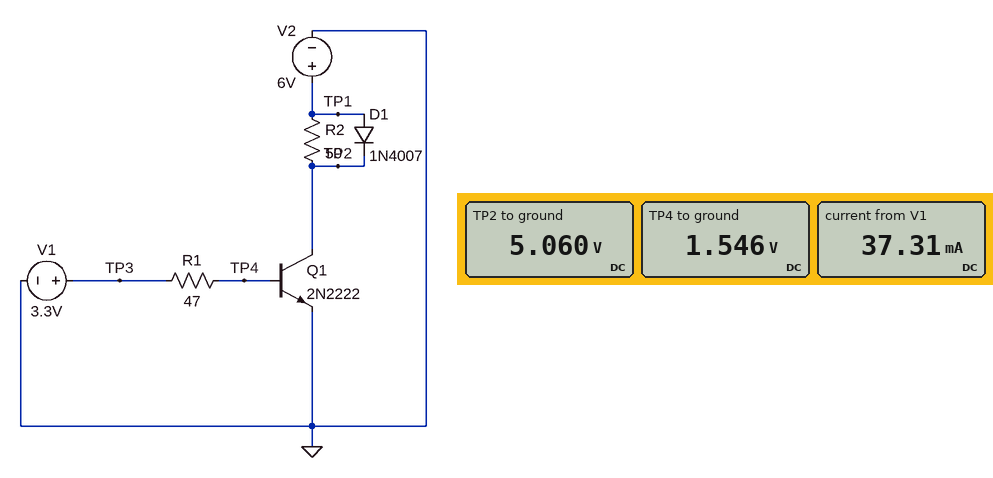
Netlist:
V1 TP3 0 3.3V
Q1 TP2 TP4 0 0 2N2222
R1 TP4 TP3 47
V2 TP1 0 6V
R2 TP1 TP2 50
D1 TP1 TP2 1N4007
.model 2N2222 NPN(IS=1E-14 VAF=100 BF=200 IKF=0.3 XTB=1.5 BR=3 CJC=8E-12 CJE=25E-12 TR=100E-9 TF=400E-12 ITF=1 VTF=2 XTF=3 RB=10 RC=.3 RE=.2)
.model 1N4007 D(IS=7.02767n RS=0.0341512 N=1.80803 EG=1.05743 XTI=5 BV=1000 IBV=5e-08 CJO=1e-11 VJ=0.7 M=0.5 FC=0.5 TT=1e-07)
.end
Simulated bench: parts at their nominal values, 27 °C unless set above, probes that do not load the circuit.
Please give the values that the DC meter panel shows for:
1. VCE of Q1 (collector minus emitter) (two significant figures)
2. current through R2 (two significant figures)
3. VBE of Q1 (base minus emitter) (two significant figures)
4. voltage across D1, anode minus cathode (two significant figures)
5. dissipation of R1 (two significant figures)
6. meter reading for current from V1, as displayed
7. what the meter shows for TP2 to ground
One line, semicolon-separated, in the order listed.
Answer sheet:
5.1 V; 19 mA; 1.5 V; 940 mV; 65 mW; 37.31 mA; 5.060 V
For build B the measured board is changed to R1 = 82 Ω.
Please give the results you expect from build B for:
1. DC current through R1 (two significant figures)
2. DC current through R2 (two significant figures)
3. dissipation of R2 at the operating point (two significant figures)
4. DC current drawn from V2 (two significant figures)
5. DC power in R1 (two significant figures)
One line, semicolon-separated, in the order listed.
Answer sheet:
24 mA; 18 mA; 17 mW; 1.1 A; 47 mW
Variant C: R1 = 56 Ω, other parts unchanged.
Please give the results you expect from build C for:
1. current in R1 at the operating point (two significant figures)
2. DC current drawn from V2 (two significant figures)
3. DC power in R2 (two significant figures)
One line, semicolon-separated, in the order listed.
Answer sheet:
33 mA; 1.3 A; 17 mW
